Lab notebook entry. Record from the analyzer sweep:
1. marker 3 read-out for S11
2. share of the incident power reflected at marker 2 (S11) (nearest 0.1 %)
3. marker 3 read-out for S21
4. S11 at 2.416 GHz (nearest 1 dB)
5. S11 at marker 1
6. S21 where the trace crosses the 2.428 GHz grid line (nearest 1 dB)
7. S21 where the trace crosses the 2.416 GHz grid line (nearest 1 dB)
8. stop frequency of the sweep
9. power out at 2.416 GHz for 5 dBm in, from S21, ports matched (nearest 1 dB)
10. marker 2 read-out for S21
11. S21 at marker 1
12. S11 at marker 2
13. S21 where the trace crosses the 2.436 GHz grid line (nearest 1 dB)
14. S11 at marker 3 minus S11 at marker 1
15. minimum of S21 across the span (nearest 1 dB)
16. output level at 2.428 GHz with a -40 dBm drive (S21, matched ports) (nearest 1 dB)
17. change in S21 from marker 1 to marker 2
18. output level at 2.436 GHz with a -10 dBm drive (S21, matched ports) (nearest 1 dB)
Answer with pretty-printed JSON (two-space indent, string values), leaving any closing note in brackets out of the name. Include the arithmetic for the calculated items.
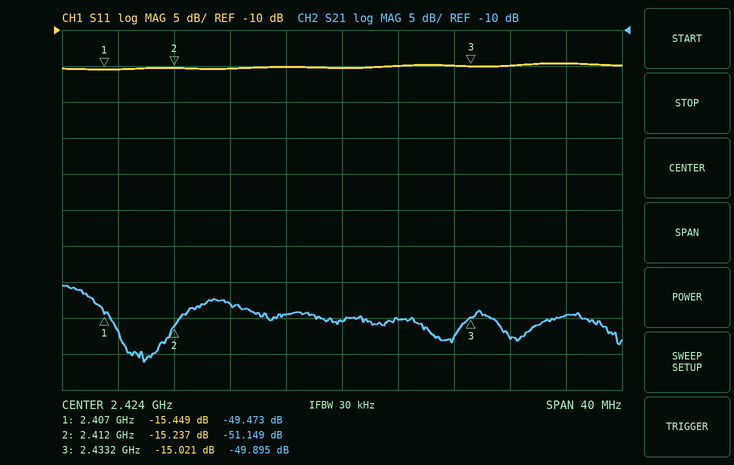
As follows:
{
  "marker 3 read-out for S11": "-15.021 dB",
  "share of the incident power reflected at marker 2 (S11)": "10^(-15.237/10) ≈ 3.0 %",
  "marker 3 read-out for S21": "-49.895 dB",
  "S11 at 2.416 GHz": "-15 dB",
  "S11 at marker 1": "-15.449 dB",
  "S21 where the trace crosses the 2.428 GHz grid line": "-50 dB",
  "S21 where the trace crosses the 2.416 GHz grid line": "-48 dB",
  "stop frequency of the sweep": "2.444 GHz",
  "power out at 2.416 GHz for 5 dBm in, from S21, ports matched": "5 dBm + (-48 dB) = -43 dBm",
  "marker 2 read-out for S21": "-51.149 dB",
  "S21 at marker 1": "-49.473 dB",
  "S11 at marker 2": "-15.237 dB",
  "S21 where the trace crosses the 2.436 GHz grid line": "-53 dB",
  "S11 at marker 3 minus S11 at marker 1": "-15.021 − (-15.449) = 0.428 dB",
  "minimum of S21 across the span": "-56 dB",
  "output level at 2.428 GHz with a -40 dBm drive (S21, matched ports)": "-40 dBm + (-50 dB) = -90 dBm",
  "change in S21 from marker 1 to marker 2": "-51.149 − (-49.473) = -1.676 dB",
  "output level at 2.436 GHz with a -10 dBm drive (S21, matched ports)": "-10 dBm + (-53 dB) = -63 dBm"
}
